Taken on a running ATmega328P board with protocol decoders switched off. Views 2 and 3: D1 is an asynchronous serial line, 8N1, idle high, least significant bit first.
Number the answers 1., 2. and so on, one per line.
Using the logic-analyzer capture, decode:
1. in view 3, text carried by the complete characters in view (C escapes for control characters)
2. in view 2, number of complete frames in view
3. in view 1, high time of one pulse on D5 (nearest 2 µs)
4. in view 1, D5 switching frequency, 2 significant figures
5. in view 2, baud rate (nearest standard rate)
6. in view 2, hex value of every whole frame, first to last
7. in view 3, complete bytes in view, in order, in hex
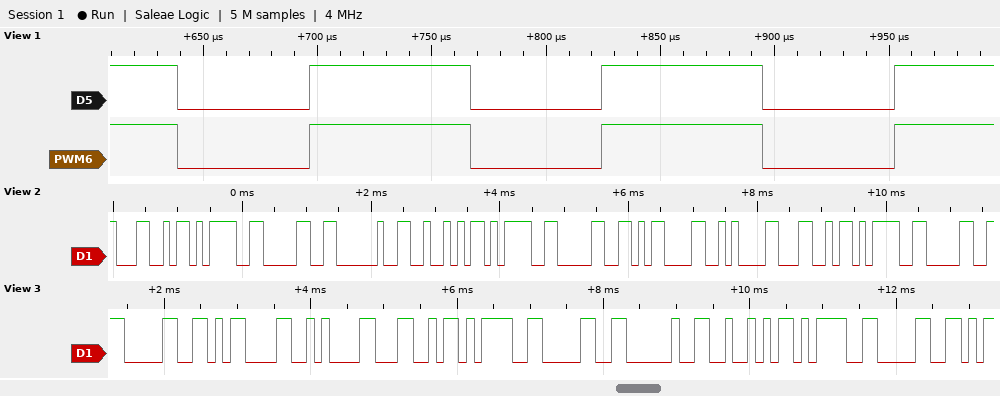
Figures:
1. "0\r\nL=0 R=0"
2. 12
3. 70 µs
4. 7.8 kHz
5. 9600 baud
6. 0x4C 0x3D 0x30 0x20 0x52 0x3D 0x30 0x0D 0x0A 0x4C 0x3D 0x30
7. 30 0D 0A 4C 3D 30 20 52 3D 30
